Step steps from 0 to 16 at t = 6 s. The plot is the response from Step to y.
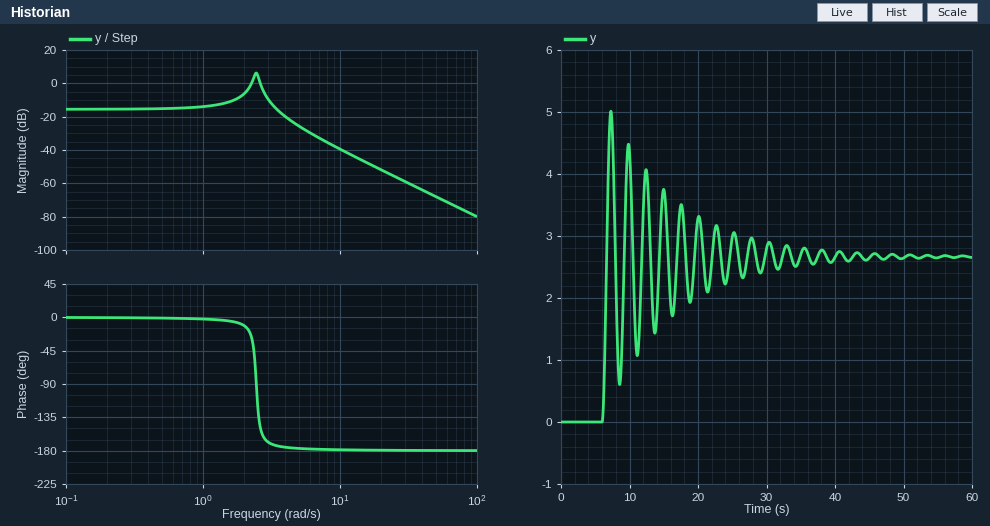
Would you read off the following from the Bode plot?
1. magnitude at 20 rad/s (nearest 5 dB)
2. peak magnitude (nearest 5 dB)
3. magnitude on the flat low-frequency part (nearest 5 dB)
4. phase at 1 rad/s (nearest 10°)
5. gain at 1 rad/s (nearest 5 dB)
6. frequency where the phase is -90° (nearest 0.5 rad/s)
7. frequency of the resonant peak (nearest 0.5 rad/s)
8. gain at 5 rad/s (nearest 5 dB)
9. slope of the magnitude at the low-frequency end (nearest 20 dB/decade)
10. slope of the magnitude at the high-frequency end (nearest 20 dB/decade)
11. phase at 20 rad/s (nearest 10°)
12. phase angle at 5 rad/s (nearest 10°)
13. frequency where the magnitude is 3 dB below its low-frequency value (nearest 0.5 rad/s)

-50 dB
5 dB
-15 dB
0°
-15 dB
2.5 rad/s
2.5 rad/s
-25 dB
0 dB/decade
-40 dB/decade
-180°
-180°
4.0 rad/s
